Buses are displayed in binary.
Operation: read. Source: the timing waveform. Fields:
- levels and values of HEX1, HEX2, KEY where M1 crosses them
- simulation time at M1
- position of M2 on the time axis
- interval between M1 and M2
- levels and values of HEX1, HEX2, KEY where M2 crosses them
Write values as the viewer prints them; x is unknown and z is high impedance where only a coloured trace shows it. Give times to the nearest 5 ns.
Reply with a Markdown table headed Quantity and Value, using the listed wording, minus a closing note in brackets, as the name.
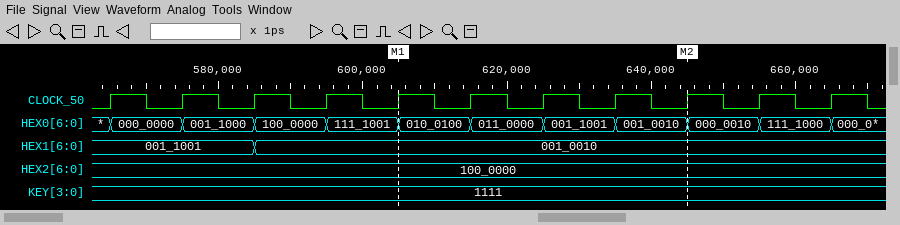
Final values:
| Quantity | Value |
|---|---|
| levels and values of HEX1, HEX2, KEY where M1 crosses them | HEX1=001_0010, HEX2=100_0000, KEY=1111 |
| simulation time at M1 | 605 ns |
| position of M2 on the time axis | 645 ns |
| interval between M1 and M2 | 40 ns |
| levels and values of HEX1, HEX2, KEY where M2 crosses them | HEX1=001_0010, HEX2=100_0000, KEY=1111 |
